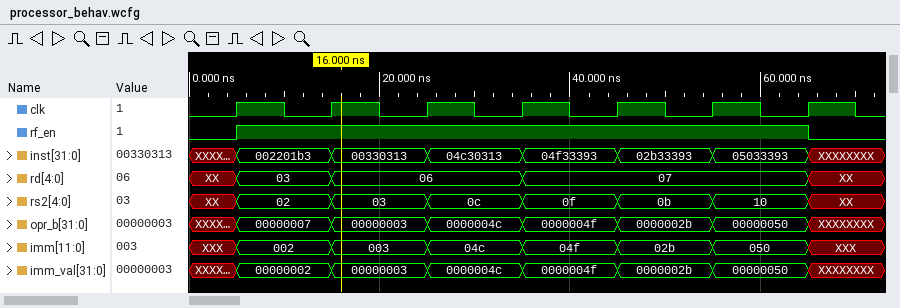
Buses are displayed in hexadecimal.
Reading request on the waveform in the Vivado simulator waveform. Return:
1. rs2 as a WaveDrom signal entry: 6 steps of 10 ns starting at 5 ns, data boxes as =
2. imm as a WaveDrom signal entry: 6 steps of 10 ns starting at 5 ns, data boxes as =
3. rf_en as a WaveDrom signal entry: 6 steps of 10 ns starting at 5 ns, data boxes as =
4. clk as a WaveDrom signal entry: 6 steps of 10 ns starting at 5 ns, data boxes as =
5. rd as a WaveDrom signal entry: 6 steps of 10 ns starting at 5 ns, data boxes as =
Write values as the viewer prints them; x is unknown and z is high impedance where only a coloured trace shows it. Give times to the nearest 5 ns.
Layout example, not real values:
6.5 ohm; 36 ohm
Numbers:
{name: 'rs2', wave: '======', data: '02 03 0c 0f 0b 10'}; {name: 'imm', wave: '======', data: '002 003 04c 04f 02b 050'}; {name: 'rf_en', wave: '1.....'}; {name: 'clk', wave: 'p.....'}; {name: 'rd', wave: '==.=..', data: '03 06 07'}
